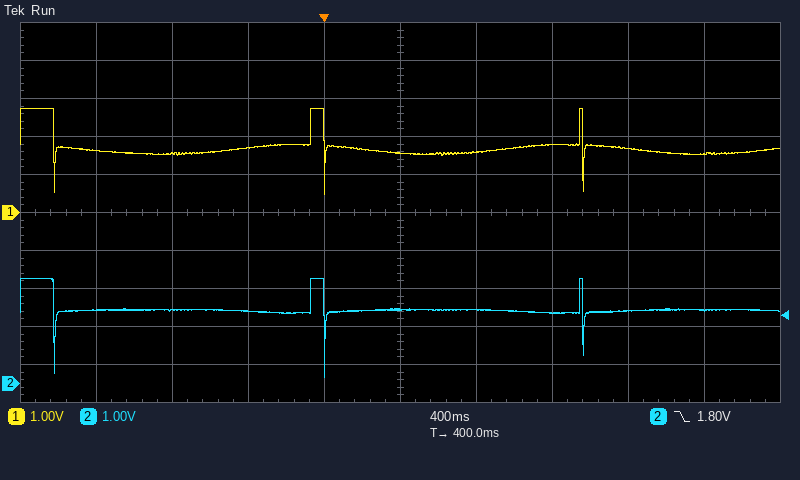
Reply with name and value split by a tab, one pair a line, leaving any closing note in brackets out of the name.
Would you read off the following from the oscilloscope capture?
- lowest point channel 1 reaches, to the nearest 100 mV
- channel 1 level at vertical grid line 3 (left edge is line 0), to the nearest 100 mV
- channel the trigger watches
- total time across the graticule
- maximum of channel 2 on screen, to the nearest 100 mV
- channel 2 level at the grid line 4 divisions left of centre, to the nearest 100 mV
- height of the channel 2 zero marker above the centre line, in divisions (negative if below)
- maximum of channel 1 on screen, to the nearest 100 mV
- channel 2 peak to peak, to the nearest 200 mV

lowest point channel 1 reaches, to the nearest 100 mV	500 mV
channel 1 level at vertical grid line 3 (left edge is line 0), to the nearest 100 mV	1.7 V
channel the trigger watches	channel 2
total time across the graticule	4 s
maximum of channel 2 on screen, to the nearest 100 mV	2.8 V
channel 2 level at the grid line 4 divisions left of centre, to the nearest 100 mV	1.9 V
height of the channel 2 zero marker above the centre line, in divisions	-4.5 div
maximum of channel 1 on screen, to the nearest 100 mV	2.7 V
channel 2 peak to peak, to the nearest 200 mV	2.6 V
